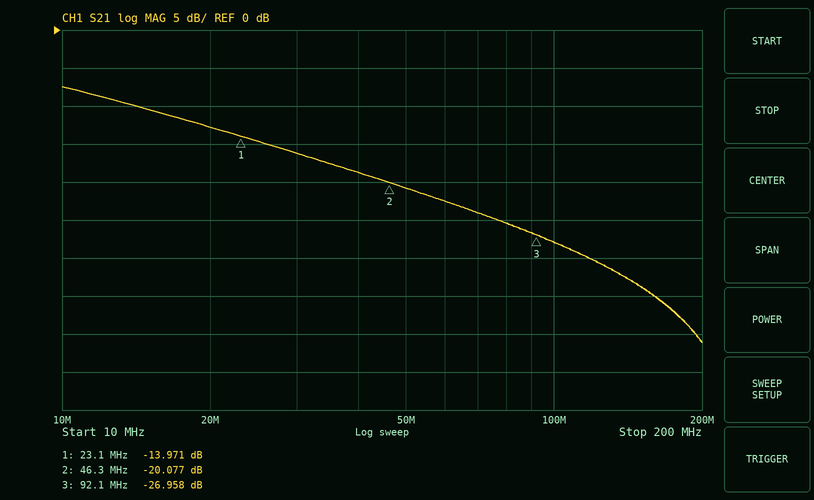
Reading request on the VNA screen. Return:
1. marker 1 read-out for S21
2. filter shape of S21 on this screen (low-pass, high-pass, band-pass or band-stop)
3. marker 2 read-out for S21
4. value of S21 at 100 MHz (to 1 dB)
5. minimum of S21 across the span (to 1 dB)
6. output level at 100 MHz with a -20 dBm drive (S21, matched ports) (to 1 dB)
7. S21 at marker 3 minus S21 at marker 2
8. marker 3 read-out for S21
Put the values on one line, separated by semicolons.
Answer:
-13.971 dB; low-pass; -20.077 dB; -28 dB; -41 dB; -48 dBm; -6.881 dB; -26.958 dB
